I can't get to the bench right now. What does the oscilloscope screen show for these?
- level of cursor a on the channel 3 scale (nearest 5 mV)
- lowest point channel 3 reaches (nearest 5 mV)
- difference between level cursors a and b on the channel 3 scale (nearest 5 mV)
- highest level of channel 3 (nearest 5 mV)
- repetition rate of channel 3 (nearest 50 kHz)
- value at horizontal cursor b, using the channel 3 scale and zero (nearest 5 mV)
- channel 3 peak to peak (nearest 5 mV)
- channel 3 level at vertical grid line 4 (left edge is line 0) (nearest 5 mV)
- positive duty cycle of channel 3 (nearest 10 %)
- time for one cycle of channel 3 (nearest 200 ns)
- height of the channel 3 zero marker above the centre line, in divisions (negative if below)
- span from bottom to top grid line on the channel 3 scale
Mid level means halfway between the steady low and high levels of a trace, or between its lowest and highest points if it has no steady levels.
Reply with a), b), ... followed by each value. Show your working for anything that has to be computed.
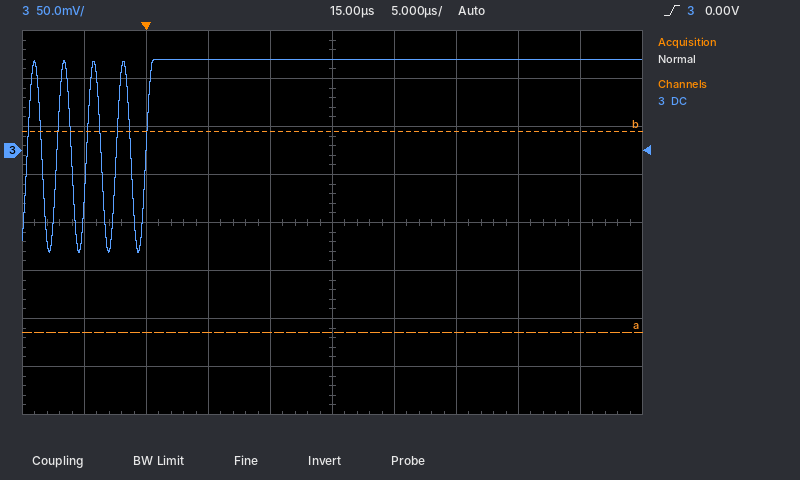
a) -190 mV
b) -105 mV
c) 210 mV
d) 95 mV
e) 1 / 2.4 µs ≈ 417 kHz, so 400 kHz to the nearest 50 kHz
f) 20 mV
g) 95 mV − (-105 mV) = 200 mV
h) 95 mV
i) 50 %
j) 2.4 µs
k) +1.5 div
l) 400 mV
